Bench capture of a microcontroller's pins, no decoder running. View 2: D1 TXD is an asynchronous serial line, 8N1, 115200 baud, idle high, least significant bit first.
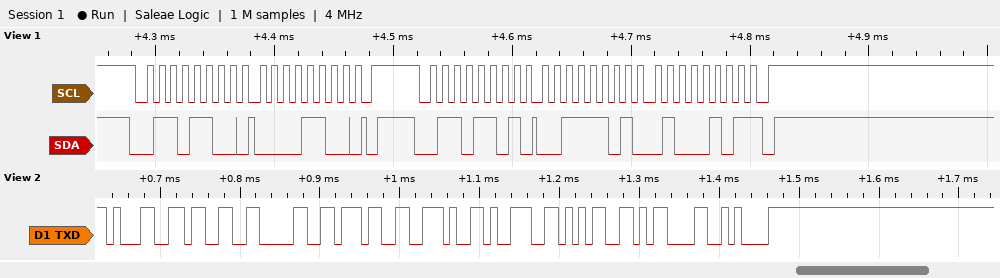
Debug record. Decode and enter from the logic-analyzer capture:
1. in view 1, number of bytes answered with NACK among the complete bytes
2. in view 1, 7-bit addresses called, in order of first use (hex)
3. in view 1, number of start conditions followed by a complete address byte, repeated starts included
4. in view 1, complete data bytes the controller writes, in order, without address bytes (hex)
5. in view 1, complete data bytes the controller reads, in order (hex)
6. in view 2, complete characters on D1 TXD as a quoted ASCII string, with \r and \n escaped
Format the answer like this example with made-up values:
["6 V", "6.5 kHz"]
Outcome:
["1", "0x36", "2", "0C", "3D 45", "\"1307.95\\r\\n\""]
